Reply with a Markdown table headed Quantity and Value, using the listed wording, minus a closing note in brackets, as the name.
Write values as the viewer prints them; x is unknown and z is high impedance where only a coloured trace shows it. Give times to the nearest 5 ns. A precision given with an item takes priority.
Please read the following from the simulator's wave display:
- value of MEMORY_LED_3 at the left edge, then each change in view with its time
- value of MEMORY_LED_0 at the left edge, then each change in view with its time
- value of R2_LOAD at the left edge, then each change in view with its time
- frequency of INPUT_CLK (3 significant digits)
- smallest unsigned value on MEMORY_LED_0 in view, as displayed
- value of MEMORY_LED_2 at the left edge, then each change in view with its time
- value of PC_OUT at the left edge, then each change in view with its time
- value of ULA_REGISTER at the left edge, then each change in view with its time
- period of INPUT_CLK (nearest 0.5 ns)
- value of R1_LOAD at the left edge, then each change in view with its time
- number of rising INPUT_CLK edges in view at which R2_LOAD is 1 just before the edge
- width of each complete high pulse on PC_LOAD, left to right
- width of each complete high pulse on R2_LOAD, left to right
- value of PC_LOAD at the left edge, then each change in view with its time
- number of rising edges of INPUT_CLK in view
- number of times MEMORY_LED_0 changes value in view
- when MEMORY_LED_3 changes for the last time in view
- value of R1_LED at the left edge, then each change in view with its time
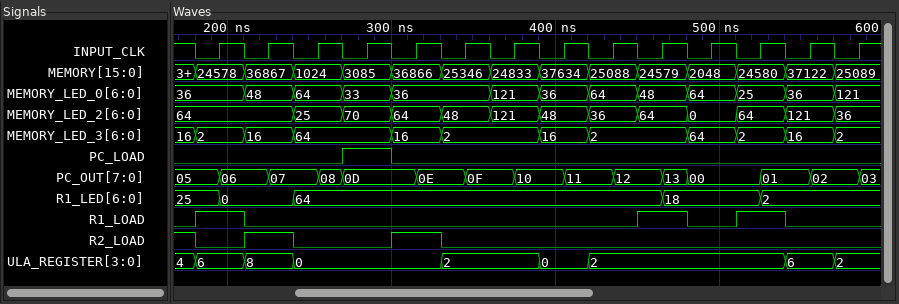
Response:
| Quantity | Value |
|---|---|
| value of MEMORY_LED_3 at the left edge, then each change in view with its time | 16, 2 at 180 ns, 16 at 210 ns, 64 at 240 ns, 16 at 300 ns, 2 at 330 ns, 16 at 390 ns, 2 at 420 ns, 64 at 480 ns, 2 at 510 ns, 16 at 540 ns, 2 at 570 ns |
| value of MEMORY_LED_0 at the left edge, then each change in view with its time | 36, 48 at 210 ns, 64 at 240 ns, 33 at 270 ns, 36 at 300 ns, 121 at 360 ns, 36 at 390 ns, 64 at 420 ns, 48 at 450 ns, 64 at 480 ns, 25 at 510 ns, 36 at 540 ns, 121 at 570 ns |
| value of R2_LOAD at the left edge, then each change in view with its time | 1, 0 at 180 ns, 1 at 210 ns, 0 at 240 ns, 1 at 300 ns, 0 at 330 ns |
| frequency of INPUT_CLK | 33.3 MHz |
| smallest unsigned value on MEMORY_LED_0 in view, as displayed | 25 |
| value of MEMORY_LED_2 at the left edge, then each change in view with its time | 64, 25 at 240 ns, 70 at 270 ns, 64 at 300 ns, 48 at 330 ns, 121 at 360 ns, 48 at 390 ns, 36 at 420 ns, 64 at 450 ns, 0 at 480 ns, 64 at 510 ns, 121 at 540 ns, 36 at 570 ns |
| value of PC_OUT at the left edge, then each change in view with its time | 05, 06 at 195 ns, 07 at 225 ns, 08 at 255 ns, 0D at 270 ns, 0E at 315 ns, 0F at 345 ns, 10 at 375 ns, 11 at 405 ns, 12 at 435 ns, 13 at 465 ns, 00 at 480 ns, 01 at 525 ns, 02 at 555 ns, 03 at 585 ns |
| value of ULA_REGISTER at the left edge, then each change in view with its time | 4, 6 at 180 ns, 8 at 210 ns, 0 at 240 ns, 2 at 330 ns, 0 at 390 ns, 2 at 420 ns, 6 at 540 ns, 2 at 570 ns |
| period of INPUT_CLK | 30 ns |
| value of R1_LOAD at the left edge, then each change in view with its time | 0, 1 at 180 ns, 0 at 210 ns, 1 at 450 ns, 0 at 480 ns, 1 at 510 ns, 0 at 540 ns |
| number of rising INPUT_CLK edges in view at which R2_LOAD is 1 just before the edge | 2 |
| width of each complete high pulse on PC_LOAD, left to right | 30 ns |
| width of each complete high pulse on R2_LOAD, left to right | 30 ns, 30 ns |
| value of PC_LOAD at the left edge, then each change in view with its time | 0, 1 at 270 ns, 0 at 300 ns |
| number of rising edges of INPUT_CLK in view | 14 |
| number of times MEMORY_LED_0 changes value in view | 12 |
| when MEMORY_LED_3 changes for the last time in view | 570 ns |
| value of R1_LED at the left edge, then each change in view with its time | 25, 0 at 195 ns, 64 at 240 ns, 18 at 465 ns, 2 at 525 ns |
